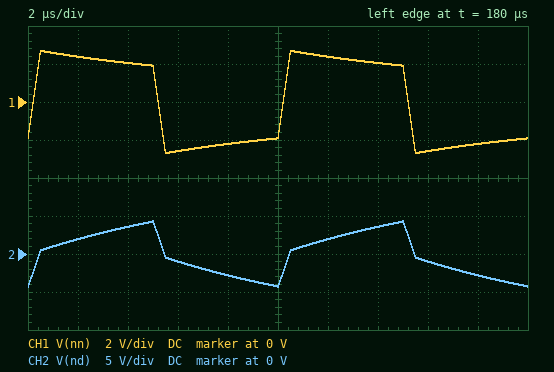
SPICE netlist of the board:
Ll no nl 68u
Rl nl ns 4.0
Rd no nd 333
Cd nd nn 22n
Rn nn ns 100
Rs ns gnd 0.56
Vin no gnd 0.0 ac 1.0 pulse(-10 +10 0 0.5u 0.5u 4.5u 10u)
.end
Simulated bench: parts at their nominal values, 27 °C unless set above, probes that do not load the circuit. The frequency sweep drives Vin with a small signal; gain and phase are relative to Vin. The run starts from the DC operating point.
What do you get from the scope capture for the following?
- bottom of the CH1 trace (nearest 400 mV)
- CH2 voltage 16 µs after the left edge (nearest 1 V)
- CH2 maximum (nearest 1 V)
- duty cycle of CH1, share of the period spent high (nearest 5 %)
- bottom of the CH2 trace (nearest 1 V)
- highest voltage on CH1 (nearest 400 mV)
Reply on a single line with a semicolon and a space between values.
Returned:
-2.8 V; -1 V; 4 V; 50 %; -4 V; 2.8 V
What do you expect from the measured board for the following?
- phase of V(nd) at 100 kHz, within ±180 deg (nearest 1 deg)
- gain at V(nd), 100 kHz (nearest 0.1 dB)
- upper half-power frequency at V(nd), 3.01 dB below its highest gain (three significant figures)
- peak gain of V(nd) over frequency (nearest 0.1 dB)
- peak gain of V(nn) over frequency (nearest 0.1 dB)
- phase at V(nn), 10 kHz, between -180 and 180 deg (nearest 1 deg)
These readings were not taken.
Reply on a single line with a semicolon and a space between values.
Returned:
-28 deg; -10.8 dB; 19.5 kHz; 0 dB; -12.7 dB; 18 deg
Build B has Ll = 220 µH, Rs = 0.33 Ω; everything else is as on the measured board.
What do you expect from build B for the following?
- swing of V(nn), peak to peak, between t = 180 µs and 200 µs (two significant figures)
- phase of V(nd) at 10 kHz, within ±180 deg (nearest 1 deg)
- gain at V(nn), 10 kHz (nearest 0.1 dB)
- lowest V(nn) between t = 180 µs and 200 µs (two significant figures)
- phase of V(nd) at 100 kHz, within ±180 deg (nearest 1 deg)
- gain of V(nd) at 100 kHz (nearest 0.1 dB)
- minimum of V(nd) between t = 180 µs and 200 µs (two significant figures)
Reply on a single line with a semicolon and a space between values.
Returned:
5.6 V; -23 deg; -19.7 dB; -2.8 V; -27 deg; -11.0 dB; -4.2 V
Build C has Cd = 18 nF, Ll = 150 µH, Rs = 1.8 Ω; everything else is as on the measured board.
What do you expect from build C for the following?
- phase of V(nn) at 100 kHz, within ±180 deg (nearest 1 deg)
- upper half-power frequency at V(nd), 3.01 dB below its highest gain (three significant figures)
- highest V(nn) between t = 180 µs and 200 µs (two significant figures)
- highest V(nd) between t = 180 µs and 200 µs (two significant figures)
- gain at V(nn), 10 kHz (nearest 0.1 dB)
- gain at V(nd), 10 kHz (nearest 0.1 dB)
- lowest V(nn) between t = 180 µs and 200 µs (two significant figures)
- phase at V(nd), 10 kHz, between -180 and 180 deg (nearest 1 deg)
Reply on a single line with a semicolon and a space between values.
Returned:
8 deg; 24.3 kHz; 2.8 V; 4.7 V; -18.2 dB; -0.4 dB; -2.8 V; -18 deg
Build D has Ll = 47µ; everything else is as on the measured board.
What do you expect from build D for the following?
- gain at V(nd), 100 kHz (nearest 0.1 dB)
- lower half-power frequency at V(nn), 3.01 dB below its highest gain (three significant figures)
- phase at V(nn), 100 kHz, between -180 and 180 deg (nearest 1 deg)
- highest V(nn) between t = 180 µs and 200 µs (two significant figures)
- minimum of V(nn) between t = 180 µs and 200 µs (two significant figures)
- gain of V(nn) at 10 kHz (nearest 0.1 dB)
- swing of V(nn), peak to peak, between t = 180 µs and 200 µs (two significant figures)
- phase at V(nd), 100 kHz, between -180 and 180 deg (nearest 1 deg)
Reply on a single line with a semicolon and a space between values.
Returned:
-10.7 dB; 15.5 kHz; 6 deg; 2.6 V; -2.6 V; -16.9 dB; 5.3 V; -28 deg
